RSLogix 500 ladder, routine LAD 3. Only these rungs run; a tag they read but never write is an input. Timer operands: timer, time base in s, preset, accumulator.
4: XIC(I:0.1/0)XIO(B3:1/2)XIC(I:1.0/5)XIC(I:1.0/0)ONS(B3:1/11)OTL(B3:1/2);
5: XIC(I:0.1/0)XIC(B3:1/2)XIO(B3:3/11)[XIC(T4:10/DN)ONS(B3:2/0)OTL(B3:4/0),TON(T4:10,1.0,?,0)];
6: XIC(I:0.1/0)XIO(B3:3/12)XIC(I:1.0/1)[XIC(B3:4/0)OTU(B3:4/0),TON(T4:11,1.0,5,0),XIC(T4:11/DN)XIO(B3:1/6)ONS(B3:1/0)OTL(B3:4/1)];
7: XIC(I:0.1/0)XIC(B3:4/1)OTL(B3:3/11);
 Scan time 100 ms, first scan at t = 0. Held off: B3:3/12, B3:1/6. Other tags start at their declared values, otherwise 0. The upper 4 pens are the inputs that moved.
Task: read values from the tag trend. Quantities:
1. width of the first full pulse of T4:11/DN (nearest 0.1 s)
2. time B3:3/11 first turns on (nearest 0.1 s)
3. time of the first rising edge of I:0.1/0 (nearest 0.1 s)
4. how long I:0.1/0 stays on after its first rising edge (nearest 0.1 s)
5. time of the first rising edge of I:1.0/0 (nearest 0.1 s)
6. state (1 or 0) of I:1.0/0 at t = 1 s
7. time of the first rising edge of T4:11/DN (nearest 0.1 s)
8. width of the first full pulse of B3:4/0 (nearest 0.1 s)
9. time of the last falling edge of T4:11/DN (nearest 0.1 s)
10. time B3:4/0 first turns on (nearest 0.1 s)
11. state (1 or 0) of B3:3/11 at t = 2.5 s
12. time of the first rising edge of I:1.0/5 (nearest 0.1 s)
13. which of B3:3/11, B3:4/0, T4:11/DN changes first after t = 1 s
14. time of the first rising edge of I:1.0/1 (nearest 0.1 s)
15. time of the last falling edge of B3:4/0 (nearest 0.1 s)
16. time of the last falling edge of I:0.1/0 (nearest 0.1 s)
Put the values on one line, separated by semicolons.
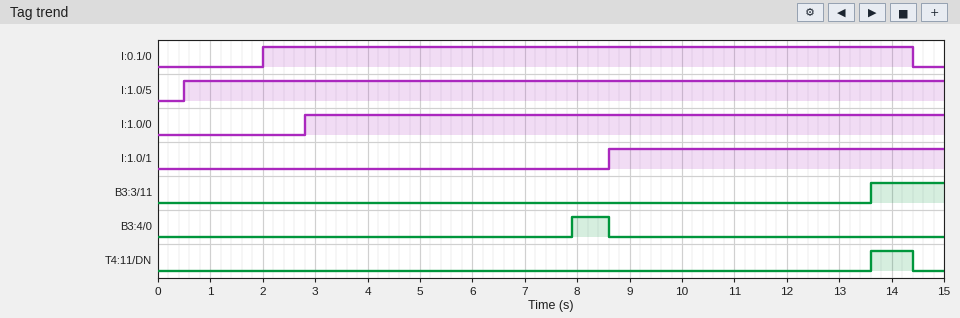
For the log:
0.8 s; 13.6 s; 2.0 s; 12.4 s; 2.8 s; 0; 13.6 s; 0.7 s; 14.4 s; 7.9 s; 0; 0.5 s; B3:4/0; 8.6 s; 8.6 s; 14.4 s
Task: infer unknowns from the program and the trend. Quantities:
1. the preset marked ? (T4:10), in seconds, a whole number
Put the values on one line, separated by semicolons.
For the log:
5 s
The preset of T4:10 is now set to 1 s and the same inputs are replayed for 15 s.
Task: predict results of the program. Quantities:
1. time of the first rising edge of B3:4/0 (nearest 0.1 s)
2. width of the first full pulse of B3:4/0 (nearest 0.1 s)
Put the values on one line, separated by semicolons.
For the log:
3.9 s; 4.7 s
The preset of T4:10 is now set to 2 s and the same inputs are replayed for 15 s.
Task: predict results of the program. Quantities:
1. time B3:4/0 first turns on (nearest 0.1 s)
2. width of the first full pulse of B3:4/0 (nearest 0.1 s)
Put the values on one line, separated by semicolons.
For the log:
4.9 s; 3.7 s
